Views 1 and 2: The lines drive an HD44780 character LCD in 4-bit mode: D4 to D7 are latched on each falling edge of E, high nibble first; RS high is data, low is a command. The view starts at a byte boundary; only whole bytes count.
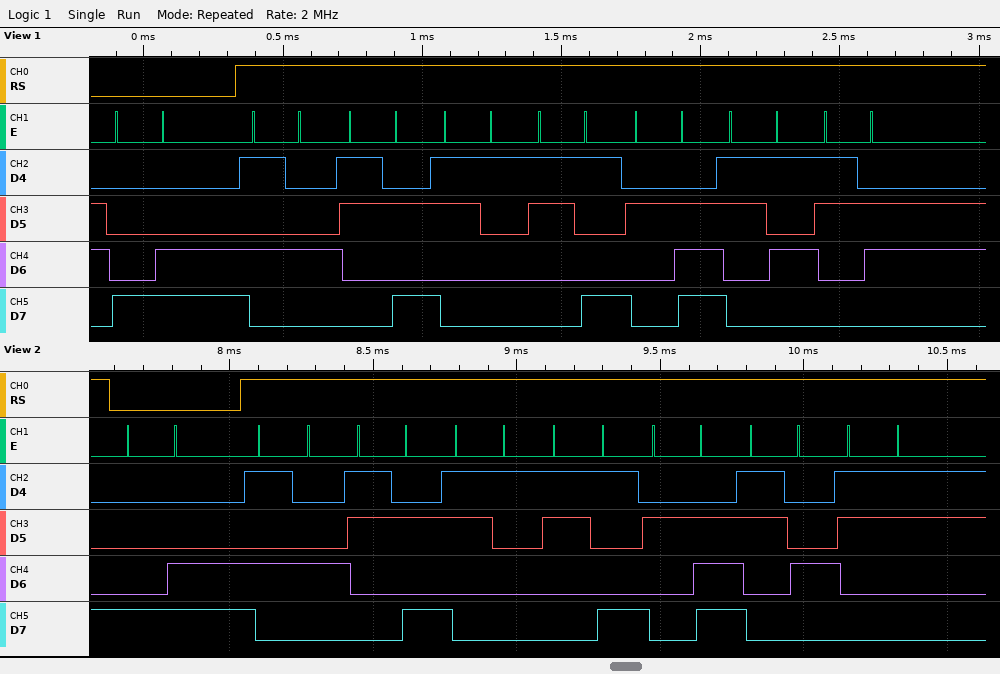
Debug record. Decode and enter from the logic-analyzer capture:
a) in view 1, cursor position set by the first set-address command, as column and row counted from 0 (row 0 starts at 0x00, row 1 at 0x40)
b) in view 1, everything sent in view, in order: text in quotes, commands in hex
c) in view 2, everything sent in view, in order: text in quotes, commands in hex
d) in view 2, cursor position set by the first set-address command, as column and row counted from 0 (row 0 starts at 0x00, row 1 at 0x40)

column 12, row 0
0x8C "T:19.56"
0x8C "T:19.43"
column 12, row 0
